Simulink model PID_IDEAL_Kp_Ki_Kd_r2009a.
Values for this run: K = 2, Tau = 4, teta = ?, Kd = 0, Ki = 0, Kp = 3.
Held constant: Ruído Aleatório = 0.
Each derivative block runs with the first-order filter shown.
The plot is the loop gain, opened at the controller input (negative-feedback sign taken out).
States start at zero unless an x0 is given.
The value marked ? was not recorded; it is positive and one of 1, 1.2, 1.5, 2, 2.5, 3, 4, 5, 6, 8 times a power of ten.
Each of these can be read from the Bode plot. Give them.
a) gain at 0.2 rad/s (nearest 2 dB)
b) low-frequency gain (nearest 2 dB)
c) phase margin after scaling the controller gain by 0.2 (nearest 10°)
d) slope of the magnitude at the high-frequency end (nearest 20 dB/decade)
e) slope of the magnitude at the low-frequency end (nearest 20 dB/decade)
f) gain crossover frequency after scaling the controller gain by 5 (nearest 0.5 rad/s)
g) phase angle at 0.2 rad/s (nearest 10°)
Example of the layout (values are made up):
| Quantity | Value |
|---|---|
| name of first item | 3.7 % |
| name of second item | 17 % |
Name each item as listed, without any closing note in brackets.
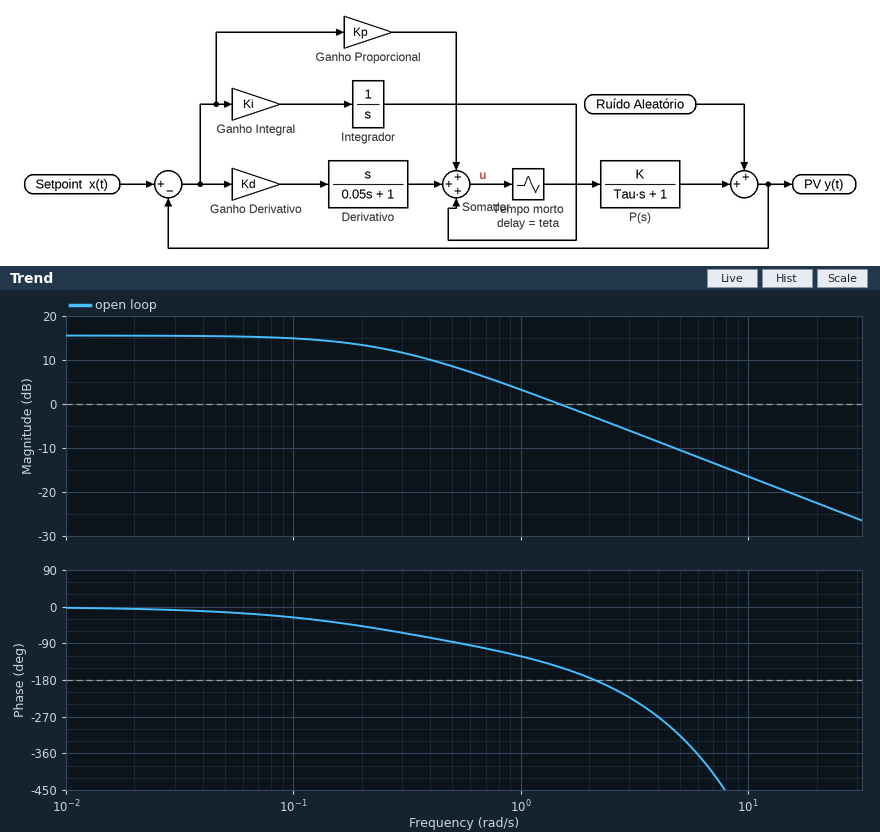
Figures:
| Quantity | Value |
|---|---|
| gain at 0.2 rad/s | 14 dB |
| low-frequency gain | 16 dB |
| phase margin after scaling the controller gain by 0.2 | 140° |
| slope of the magnitude at the high-frequency end | -20 dB/decade |
| slope of the magnitude at the low-frequency end | 0 dB/decade |
| gain crossover frequency after scaling the controller gain by 5 | 7.5 rad/s |
| phase angle at 0.2 rad/s | -50° |
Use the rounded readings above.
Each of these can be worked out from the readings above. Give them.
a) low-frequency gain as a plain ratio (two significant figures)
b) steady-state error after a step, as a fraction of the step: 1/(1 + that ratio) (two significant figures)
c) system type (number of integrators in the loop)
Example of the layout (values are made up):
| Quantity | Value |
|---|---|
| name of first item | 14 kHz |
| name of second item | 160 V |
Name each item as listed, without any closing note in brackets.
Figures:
| Quantity | Value |
|---|---|
| low-frequency gain as a plain ratio | 6.3 |
| steady-state error after a step, as a fraction of the step: 1/(1 + that ratio) | 0.14 |
| system type | 0 |
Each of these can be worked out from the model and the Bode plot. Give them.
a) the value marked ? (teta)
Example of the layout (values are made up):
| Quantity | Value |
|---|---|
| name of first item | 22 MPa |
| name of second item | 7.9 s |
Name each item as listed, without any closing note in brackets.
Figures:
| Quantity | Value |
|---|---|
| the value marked ? | 0.8 |
